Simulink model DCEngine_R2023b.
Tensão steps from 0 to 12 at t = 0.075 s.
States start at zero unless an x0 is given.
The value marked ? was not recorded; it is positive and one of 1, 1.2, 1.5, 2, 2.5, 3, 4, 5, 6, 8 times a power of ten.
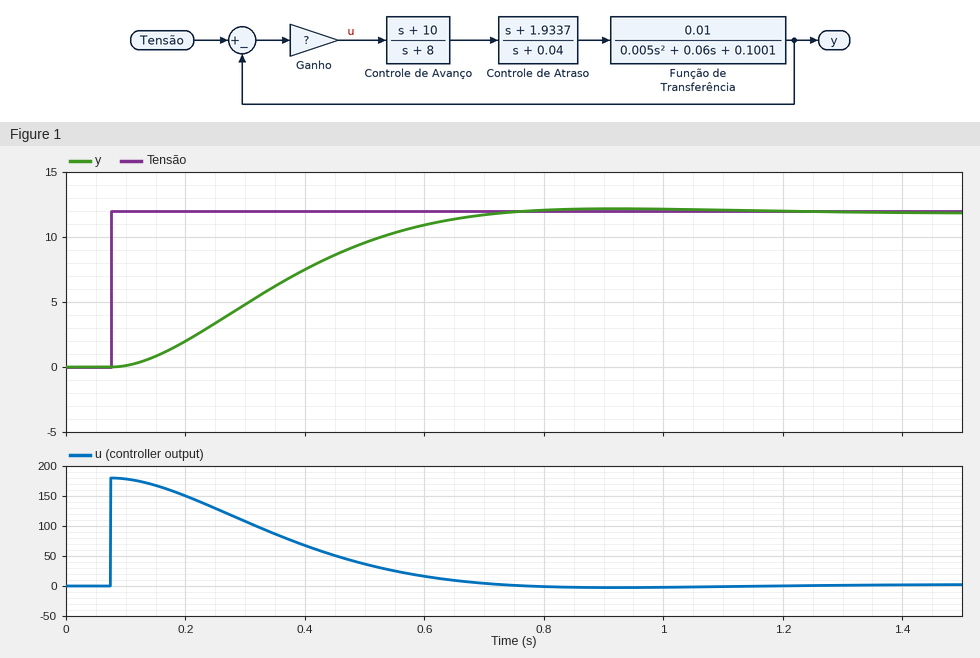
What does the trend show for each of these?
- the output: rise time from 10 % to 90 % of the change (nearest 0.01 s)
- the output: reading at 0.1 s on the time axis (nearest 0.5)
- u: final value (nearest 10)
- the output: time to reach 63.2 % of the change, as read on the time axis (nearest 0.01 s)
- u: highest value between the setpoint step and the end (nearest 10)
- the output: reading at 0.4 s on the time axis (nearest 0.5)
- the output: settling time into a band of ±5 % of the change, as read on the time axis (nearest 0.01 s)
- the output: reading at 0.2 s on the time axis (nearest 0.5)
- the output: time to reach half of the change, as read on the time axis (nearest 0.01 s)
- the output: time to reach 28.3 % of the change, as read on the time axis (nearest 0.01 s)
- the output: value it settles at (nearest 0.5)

0.41 s
0.0
0
0.40 s
180
7.5
0.64 s
2.0
0.34 s
0.25 s
12.0
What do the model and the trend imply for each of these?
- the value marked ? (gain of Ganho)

15
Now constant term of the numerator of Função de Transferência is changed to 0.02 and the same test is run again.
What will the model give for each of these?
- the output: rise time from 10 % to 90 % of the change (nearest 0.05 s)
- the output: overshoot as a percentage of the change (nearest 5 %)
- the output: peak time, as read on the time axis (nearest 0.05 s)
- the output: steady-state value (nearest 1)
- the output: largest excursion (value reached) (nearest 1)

0.20 s
15 %
0.55 s
12
14
